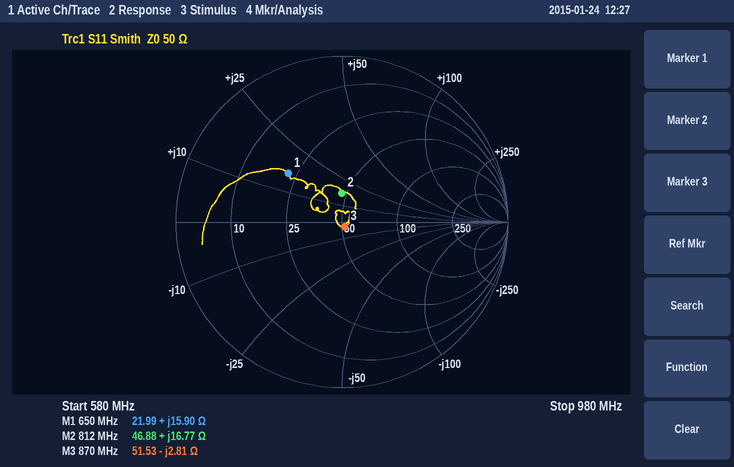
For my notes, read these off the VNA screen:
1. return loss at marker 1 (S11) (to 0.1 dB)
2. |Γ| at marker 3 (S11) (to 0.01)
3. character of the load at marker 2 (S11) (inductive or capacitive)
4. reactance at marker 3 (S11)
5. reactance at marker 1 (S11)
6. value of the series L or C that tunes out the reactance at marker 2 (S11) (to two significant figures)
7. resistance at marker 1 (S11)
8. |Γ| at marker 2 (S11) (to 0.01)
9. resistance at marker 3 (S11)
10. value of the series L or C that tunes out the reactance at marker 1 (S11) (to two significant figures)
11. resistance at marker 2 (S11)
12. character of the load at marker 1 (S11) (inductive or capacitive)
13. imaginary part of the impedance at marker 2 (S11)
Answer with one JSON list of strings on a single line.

["7.2 dB", "0.03", "inductive", "-2.81 Ω", "+15.90 Ω", "12 pF", "21.99 Ω", "0.17", "51.53 Ω", "15 pF", "46.88 Ω", "inductive", "+16.77 Ω"]
